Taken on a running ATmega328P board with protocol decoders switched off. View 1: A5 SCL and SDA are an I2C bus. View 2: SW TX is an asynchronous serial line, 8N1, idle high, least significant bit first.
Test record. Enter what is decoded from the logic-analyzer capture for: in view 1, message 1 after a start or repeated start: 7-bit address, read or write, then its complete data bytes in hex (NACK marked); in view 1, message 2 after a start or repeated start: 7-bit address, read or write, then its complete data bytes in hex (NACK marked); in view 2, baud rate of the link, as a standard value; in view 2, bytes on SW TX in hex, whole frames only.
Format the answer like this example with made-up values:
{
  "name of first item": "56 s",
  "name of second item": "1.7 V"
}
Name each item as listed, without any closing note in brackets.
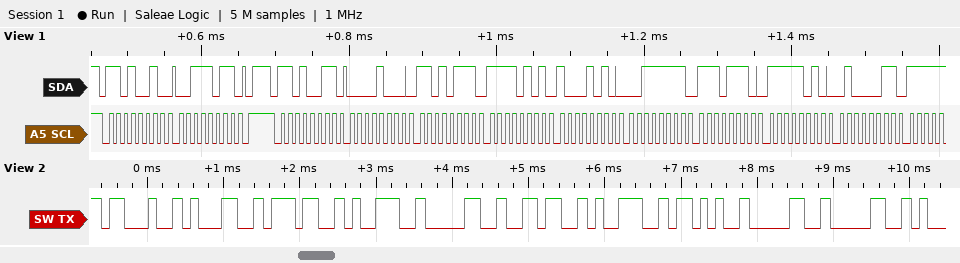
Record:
{
  "in view 1, message 1 after a start or repeated start: 7-bit address, read or write, then its complete data bytes in hex": "0x69 write: 3B",
  "in view 1, message 2 after a start or repeated start: 7-bit address, read or write, then its complete data bytes in hex": "0x69 read: 08 D7 F5 8A 3F EE FA 43",
  "in view 2, baud rate of the link, as a standard value": "9600 baud",
  "in view 2, bytes on SW TX in hex, whole frames only": "23 31 37 39 30 36 39 2B 30 30"
}
